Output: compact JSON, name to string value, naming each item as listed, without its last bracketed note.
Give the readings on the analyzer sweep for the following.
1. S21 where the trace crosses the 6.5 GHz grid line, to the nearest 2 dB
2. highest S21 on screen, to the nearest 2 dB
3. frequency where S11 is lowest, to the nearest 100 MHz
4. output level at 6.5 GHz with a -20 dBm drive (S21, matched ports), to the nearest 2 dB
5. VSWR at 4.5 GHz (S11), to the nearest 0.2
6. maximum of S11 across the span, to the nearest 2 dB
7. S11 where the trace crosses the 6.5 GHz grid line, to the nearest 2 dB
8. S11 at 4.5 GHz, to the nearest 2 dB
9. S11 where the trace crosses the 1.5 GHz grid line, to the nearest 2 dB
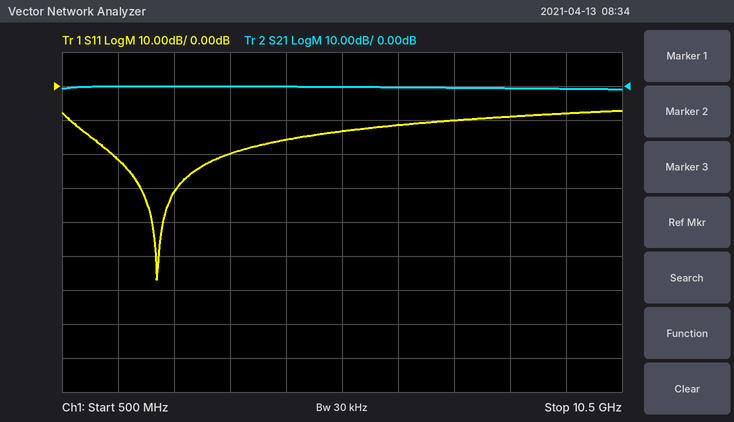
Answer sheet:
{"S21 where the trace crosses the 6.5 GHz grid line, to the nearest 2 dB": "0 dB", "highest S21 on screen, to the nearest 2 dB": "0 dB", "frequency where S11 is lowest, to the nearest 100 MHz": "2.2 GHz", "output level at 6.5 GHz with a -20 dBm drive (S21, matched ports), to the nearest 2 dB": "-20 dBm", "VSWR at 4.5 GHz (S11), to the nearest 0.2": "1.4", "maximum of S11 across the span, to the nearest 2 dB": "-8 dB", "S11 where the trace crosses the 6.5 GHz grid line, to the nearest 2 dB": "-12 dB", "S11 at 4.5 GHz, to the nearest 2 dB": "-16 dB", "S11 where the trace crosses the 1.5 GHz grid line, to the nearest 2 dB": "-22 dB"}
